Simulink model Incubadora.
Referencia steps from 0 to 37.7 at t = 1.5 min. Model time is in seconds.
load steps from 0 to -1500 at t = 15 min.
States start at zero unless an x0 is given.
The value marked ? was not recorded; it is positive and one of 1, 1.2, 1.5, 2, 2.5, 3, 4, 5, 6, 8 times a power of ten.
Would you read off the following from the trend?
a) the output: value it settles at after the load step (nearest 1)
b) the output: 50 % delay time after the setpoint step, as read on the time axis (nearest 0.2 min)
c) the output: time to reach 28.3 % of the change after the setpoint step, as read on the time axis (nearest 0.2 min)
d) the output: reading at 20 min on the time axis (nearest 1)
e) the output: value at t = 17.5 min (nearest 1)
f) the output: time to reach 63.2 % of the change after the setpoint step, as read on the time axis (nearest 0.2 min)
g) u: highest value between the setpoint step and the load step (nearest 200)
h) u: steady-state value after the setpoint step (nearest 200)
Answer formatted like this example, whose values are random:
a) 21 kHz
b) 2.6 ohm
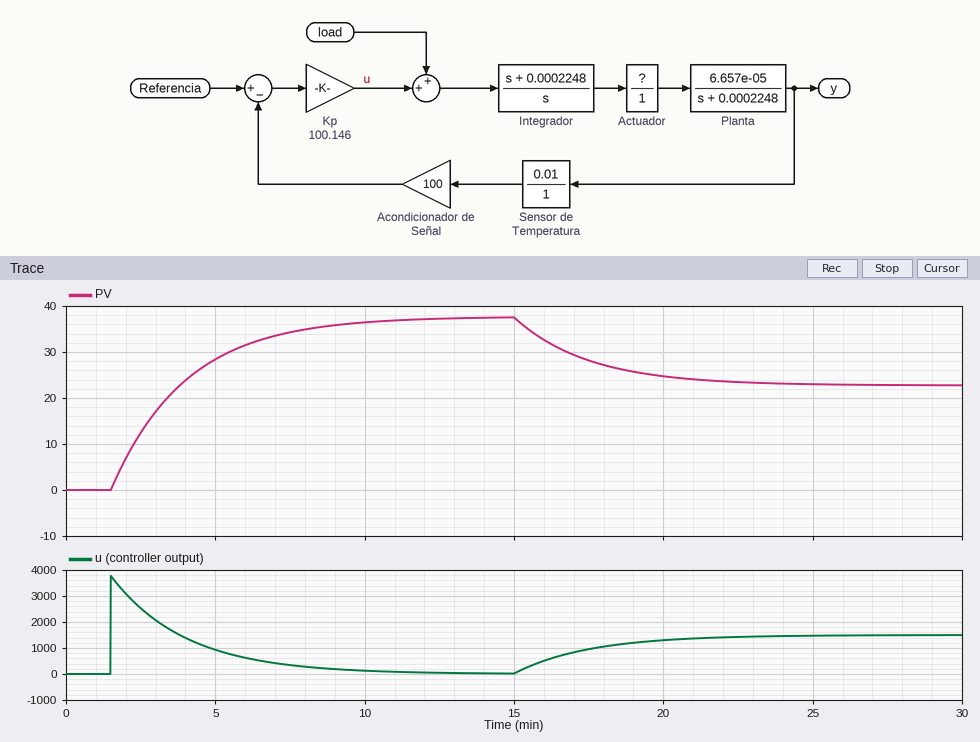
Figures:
a) 23
b) 3.2 min
c) 2.4 min
d) 25
e) 28
f) 4.0 min
g) 3800
h) 0
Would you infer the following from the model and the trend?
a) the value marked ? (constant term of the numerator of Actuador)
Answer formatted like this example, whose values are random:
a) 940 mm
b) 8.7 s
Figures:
a) 1
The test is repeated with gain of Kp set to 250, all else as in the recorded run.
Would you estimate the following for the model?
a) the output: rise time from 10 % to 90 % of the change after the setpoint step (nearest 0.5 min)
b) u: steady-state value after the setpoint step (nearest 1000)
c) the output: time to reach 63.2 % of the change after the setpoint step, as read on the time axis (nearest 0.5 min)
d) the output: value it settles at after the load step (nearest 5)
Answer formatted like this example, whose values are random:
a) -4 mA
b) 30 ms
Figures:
a) 2.0 min
b) 0
c) 2.5 min
d) 30
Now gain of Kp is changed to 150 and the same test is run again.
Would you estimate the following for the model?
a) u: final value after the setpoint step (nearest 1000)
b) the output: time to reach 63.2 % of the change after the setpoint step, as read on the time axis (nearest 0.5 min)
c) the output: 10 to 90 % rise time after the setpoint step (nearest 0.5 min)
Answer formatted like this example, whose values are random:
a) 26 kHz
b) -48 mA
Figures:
a) 0
b) 3.0 min
c) 3.5 min
